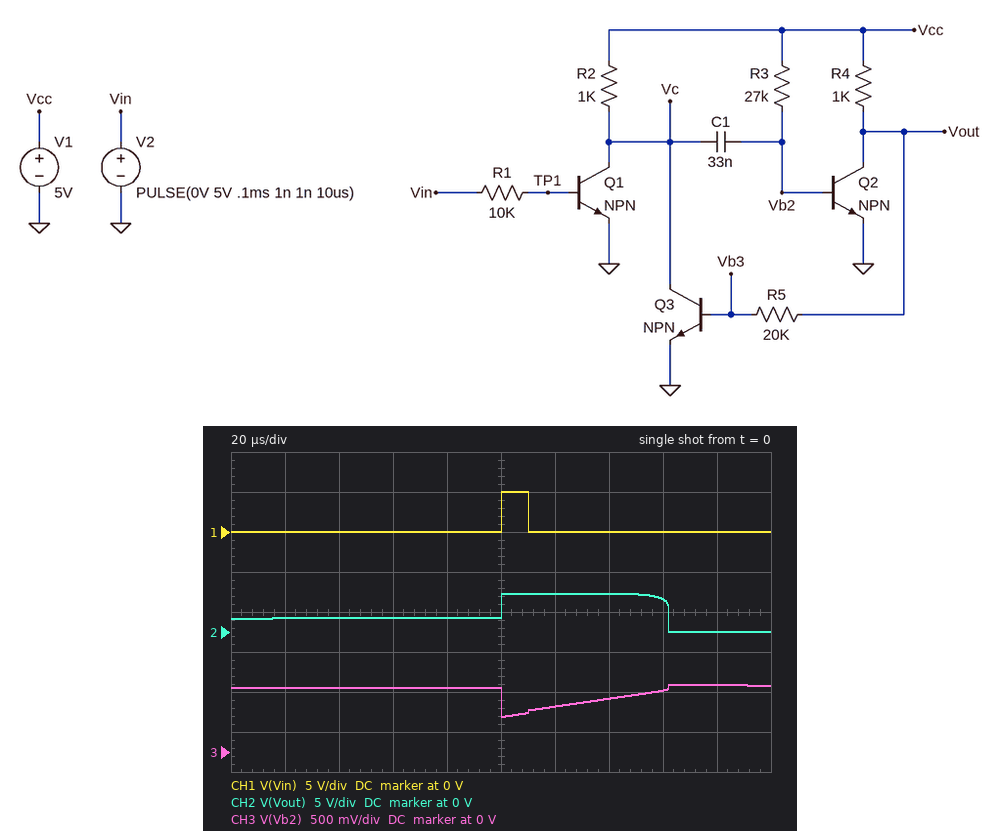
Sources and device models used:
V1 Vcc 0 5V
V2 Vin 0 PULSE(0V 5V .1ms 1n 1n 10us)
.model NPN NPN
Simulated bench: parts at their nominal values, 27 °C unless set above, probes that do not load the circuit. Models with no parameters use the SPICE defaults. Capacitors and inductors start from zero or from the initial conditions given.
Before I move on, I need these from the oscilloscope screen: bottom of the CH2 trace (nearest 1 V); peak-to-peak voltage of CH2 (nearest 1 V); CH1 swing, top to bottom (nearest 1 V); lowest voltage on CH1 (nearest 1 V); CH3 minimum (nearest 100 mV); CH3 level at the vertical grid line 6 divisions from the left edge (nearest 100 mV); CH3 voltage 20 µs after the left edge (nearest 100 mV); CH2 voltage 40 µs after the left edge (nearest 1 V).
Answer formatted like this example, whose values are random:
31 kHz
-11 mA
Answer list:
0 V
5 V
5 V
0 V
400 mV
600 mV
800 mV
2 V
